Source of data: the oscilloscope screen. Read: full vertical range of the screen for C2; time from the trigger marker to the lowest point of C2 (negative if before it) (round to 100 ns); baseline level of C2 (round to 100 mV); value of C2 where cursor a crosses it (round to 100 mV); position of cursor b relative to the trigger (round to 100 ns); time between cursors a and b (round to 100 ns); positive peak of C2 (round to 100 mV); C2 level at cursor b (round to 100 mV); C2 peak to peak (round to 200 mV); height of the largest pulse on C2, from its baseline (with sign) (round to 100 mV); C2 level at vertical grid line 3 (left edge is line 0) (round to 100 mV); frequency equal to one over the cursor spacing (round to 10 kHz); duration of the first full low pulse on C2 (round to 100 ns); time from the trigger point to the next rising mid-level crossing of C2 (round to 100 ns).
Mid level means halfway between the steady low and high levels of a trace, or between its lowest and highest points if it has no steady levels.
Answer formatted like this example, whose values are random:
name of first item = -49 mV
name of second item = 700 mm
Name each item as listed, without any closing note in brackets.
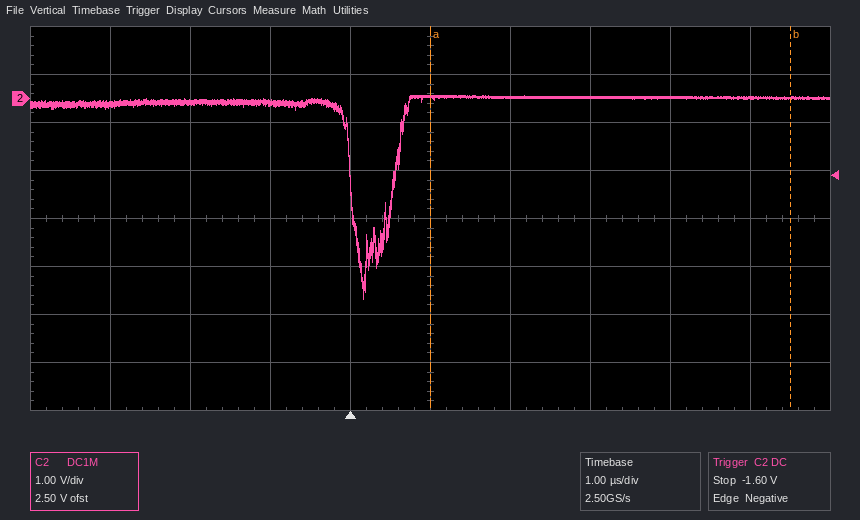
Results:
full vertical range of the screen for C2 = 8 V
time from the trigger marker to the lowest point of C2 (negative if before it) = +200 ns
baseline level of C2 = 0.0 V
value of C2 where cursor a crosses it = 0.0 V
position of cursor b relative to the trigger = +5.5 µs
time between cursors a and b = 4.5 µs
positive peak of C2 = 100 mV
C2 level at cursor b = 0.0 V
C2 peak to peak = 4.2 V
height of the largest pulse on C2, from its baseline (with sign) = -4.2 V
C2 level at vertical grid line 3 (left edge is line 0) = -100 mV
frequency equal to one over the cursor spacing = 220 kHz
duration of the first full low pulse on C2 = 500 ns
time from the trigger point to the next rising mid-level crossing of C2 = 500 ns
